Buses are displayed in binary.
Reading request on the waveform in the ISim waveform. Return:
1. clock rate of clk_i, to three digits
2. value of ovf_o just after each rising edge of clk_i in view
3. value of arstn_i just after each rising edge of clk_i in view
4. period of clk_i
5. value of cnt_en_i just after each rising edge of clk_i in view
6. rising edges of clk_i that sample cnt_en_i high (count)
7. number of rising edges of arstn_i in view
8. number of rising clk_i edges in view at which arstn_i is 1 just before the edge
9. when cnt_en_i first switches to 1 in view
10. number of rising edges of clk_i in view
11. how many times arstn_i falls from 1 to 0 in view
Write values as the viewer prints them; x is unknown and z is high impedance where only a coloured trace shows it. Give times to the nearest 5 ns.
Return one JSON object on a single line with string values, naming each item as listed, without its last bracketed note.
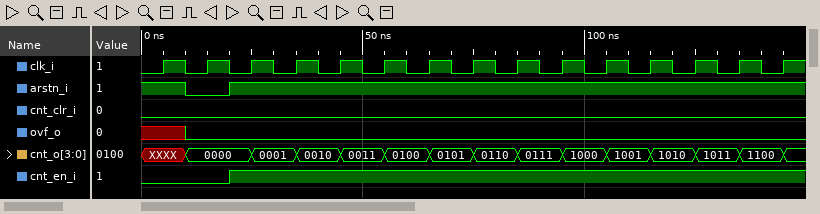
{"clock rate of clk_i, to three digits": "100 MHz", "value of ovf_o just after each rising edge of clk_i in view": "x 0 0 0 0 0 0 0 0 0 0 0 0 0 0", "value of arstn_i just after each rising edge of clk_i in view": "1 0 1 1 1 1 1 1 1 1 1 1 1 1 1", "period of clk_i": "10 ns", "value of cnt_en_i just after each rising edge of clk_i in view": "0 0 1 1 1 1 1 1 1 1 1 1 1 1 1", "rising edges of clk_i that sample cnt_en_i high": "13", "number of rising edges of arstn_i in view": "1", "number of rising clk_i edges in view at which arstn_i is 1 just before the edge": "14", "when cnt_en_i first switches to 1 in view": "20 ns", "number of rising edges of clk_i in view": "15", "how many times arstn_i falls from 1 to 0 in view": "1"}
